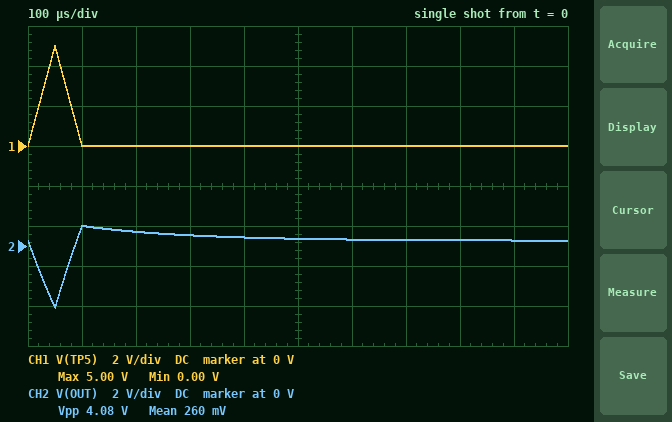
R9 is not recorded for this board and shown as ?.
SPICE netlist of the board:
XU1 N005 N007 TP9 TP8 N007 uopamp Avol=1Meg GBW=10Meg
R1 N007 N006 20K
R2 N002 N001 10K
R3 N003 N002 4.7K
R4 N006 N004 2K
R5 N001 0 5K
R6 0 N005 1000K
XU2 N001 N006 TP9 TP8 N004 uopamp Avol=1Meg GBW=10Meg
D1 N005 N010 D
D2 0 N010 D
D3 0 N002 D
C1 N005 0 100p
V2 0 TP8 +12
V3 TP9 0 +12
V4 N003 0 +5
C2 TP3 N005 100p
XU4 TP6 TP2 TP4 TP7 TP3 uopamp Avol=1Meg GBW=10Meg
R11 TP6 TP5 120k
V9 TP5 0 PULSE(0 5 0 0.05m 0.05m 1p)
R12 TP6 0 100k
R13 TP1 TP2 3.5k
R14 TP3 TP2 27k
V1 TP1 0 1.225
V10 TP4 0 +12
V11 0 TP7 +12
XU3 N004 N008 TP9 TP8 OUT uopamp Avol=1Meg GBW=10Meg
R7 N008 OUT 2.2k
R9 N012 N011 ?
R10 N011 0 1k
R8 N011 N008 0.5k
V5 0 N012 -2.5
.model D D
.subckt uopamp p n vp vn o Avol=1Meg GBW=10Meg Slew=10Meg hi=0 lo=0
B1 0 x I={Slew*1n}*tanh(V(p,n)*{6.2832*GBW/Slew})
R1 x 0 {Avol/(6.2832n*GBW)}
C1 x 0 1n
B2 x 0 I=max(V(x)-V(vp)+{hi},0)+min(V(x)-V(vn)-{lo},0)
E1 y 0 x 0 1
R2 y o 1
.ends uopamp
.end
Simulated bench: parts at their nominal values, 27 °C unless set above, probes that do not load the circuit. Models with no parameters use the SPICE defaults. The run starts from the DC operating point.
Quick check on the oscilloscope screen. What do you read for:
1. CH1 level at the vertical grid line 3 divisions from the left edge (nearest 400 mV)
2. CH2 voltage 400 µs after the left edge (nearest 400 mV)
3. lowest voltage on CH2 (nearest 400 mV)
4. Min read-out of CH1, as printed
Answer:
0 V
400 mV
-3.2 V
0.00 V
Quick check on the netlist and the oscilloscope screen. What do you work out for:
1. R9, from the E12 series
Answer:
390 Ω
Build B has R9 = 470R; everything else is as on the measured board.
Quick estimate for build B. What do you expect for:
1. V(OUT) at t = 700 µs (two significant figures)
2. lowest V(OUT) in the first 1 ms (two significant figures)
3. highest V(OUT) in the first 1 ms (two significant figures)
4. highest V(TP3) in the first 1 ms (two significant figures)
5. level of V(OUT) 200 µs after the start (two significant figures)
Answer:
610 mV
-2.6 V
1.3 V
10 V
1.0 V
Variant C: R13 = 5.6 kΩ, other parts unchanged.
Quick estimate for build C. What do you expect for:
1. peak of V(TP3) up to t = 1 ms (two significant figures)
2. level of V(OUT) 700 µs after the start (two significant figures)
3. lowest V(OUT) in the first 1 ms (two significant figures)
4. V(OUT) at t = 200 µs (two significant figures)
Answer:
7.3 V
290 mV
-2.0 V
560 mV
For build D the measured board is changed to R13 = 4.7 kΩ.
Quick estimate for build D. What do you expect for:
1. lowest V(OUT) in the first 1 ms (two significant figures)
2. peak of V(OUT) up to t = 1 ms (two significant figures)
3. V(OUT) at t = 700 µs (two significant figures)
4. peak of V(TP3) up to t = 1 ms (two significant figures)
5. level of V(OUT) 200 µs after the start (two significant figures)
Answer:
-2.3 V
830 mV
290 mV
8.3 V
610 mV
